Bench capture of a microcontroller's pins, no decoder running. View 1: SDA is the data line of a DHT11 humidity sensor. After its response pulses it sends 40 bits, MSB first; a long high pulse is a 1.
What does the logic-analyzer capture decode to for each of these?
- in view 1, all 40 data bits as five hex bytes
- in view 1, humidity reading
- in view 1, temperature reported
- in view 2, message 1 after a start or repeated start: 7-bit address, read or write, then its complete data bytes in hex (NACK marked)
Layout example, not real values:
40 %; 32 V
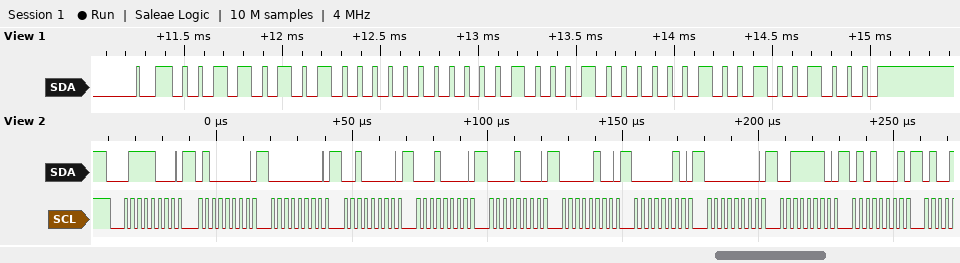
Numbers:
35 00 11 02 48; 53 %; 17.2 °C; 0x3C write: 40 00 20 10 08 04 02 00 3E 51
